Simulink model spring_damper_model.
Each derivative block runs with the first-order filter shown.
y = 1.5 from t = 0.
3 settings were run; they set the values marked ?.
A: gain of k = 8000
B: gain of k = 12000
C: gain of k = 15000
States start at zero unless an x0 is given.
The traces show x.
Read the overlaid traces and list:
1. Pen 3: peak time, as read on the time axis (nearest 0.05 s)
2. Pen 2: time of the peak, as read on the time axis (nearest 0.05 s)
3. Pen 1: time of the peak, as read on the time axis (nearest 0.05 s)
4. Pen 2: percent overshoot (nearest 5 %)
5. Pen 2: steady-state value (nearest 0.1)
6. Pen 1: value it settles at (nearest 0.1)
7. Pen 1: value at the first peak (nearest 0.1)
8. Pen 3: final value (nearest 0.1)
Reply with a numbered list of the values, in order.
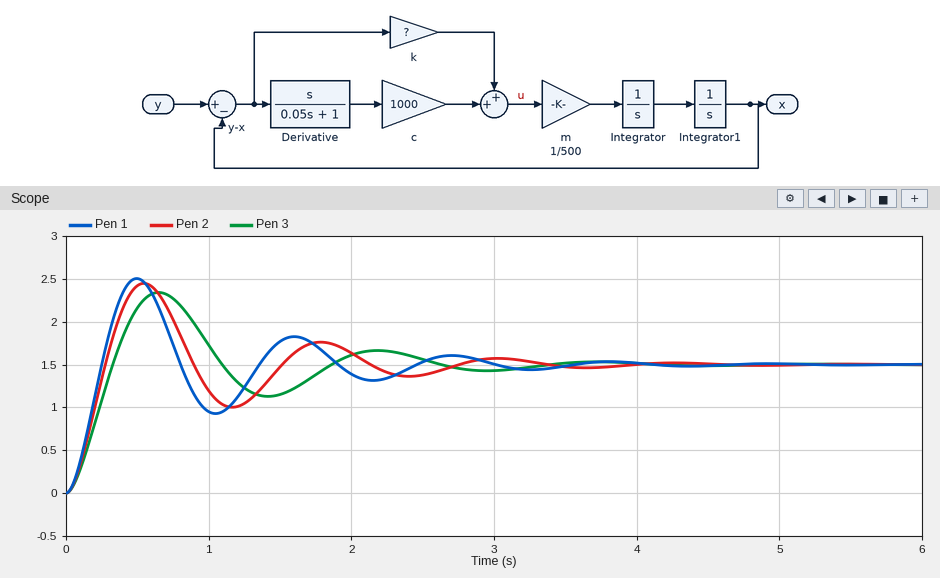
1. 0.65 s
2. 0.55 s
3. 0.50 s
4. 65 %
5. 1.5
6. 1.5
7. 2.5
8. 1.5
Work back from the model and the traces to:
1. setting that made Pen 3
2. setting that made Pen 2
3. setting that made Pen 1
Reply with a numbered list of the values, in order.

1. A
2. B
3. C
